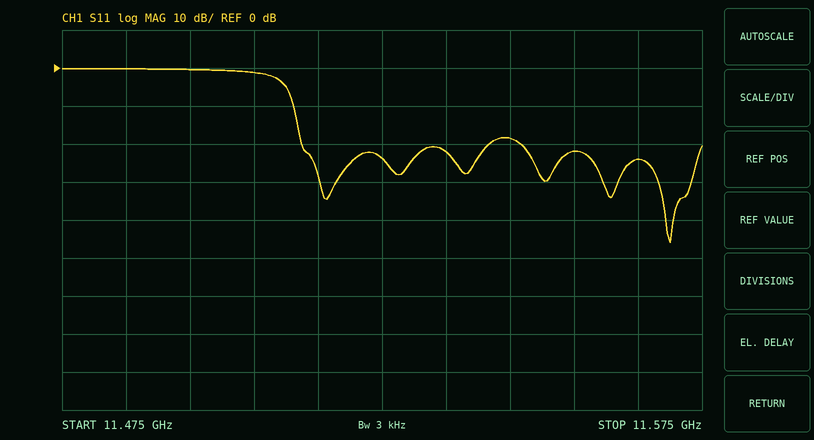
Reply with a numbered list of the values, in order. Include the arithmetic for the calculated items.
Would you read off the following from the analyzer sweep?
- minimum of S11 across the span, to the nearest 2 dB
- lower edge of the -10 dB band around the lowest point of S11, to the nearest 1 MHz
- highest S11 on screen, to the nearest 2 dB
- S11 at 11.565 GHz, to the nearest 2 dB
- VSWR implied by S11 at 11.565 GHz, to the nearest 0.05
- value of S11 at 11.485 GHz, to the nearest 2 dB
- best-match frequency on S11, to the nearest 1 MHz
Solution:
1. -46 dB
2. 11.511 GHz
3. 0 dB
4. -24 dB
5. |Γ| = 10^(-24/20) = 0.0631; VSWR = (1 + 0.0631)/(1 − 0.0631) ≈ 1.13, so 1.15 to the nearest 0.05
6. 0 dB
7. 11.570 GHz
